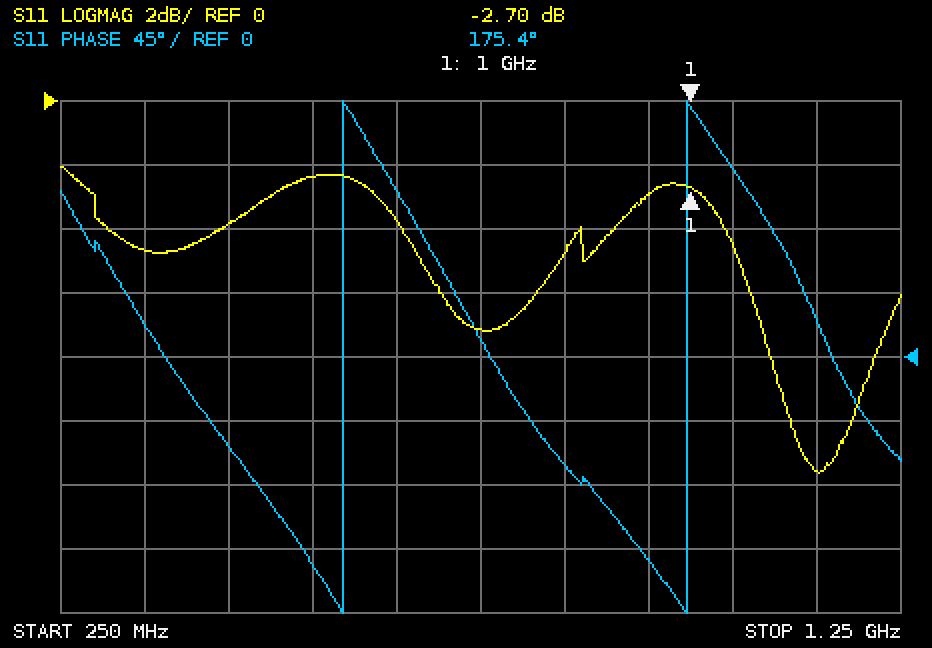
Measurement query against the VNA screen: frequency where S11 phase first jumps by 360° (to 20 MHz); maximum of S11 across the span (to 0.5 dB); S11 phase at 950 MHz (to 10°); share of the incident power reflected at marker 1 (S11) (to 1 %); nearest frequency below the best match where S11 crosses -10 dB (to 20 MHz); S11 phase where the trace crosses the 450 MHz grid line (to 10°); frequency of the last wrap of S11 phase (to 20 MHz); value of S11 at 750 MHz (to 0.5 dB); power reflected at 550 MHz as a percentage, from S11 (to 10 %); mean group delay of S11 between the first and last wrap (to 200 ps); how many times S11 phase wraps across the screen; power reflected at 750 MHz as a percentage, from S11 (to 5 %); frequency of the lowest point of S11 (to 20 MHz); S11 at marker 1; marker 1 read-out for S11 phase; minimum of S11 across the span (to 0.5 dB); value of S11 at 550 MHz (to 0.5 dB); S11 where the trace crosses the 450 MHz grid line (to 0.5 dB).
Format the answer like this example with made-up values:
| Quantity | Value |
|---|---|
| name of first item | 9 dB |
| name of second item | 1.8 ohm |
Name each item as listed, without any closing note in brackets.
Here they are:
| Quantity | Value |
|---|---|
| frequency where S11 phase first jumps by 360° | 580 MHz |
| maximum of S11 across the span | -2.0 dB |
| S11 phase at 950 MHz | -140° |
| share of the incident power reflected at marker 1 (S11) | 54 % |
| nearest frequency below the best match where S11 crosses -10 dB | 1.12 GHz |
| S11 phase where the trace crosses the 450 MHz grid line | -60° |
| frequency of the last wrap of S11 phase | 1.00 GHz |
| value of S11 at 750 MHz | -7.0 dB |
| power reflected at 550 MHz as a percentage, from S11 | 60 % |
| mean group delay of S11 between the first and last wrap | 2.4 ns |
| how many times S11 phase wraps across the screen | 2 |
| power reflected at 750 MHz as a percentage, from S11 | 20 % |
| frequency of the lowest point of S11 | 1.16 GHz |
| S11 at marker 1 | -2.70 dB |
| marker 1 read-out for S11 phase | 175.4° |
| minimum of S11 across the span | -11.5 dB |
| value of S11 at 550 MHz | -2.5 dB |
| S11 where the trace crosses the 450 MHz grid line | -4.0 dB |
